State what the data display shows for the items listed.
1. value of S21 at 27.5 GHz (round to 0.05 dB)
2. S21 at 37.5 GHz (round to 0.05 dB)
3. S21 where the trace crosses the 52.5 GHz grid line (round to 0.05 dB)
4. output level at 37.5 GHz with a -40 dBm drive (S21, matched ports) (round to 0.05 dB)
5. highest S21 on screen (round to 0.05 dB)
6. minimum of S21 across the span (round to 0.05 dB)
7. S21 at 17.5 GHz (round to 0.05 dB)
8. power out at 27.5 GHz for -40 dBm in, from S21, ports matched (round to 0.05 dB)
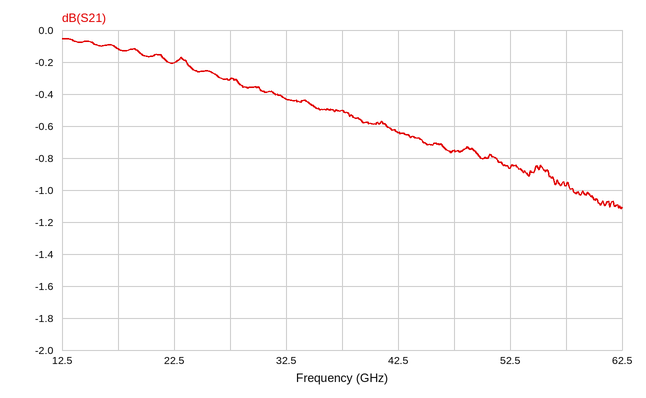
-0.30 dB
-0.50 dB
-0.85 dB
-40.50 dBm
-0.05 dB
-1.10 dB
-0.10 dB
-40.30 dBm
